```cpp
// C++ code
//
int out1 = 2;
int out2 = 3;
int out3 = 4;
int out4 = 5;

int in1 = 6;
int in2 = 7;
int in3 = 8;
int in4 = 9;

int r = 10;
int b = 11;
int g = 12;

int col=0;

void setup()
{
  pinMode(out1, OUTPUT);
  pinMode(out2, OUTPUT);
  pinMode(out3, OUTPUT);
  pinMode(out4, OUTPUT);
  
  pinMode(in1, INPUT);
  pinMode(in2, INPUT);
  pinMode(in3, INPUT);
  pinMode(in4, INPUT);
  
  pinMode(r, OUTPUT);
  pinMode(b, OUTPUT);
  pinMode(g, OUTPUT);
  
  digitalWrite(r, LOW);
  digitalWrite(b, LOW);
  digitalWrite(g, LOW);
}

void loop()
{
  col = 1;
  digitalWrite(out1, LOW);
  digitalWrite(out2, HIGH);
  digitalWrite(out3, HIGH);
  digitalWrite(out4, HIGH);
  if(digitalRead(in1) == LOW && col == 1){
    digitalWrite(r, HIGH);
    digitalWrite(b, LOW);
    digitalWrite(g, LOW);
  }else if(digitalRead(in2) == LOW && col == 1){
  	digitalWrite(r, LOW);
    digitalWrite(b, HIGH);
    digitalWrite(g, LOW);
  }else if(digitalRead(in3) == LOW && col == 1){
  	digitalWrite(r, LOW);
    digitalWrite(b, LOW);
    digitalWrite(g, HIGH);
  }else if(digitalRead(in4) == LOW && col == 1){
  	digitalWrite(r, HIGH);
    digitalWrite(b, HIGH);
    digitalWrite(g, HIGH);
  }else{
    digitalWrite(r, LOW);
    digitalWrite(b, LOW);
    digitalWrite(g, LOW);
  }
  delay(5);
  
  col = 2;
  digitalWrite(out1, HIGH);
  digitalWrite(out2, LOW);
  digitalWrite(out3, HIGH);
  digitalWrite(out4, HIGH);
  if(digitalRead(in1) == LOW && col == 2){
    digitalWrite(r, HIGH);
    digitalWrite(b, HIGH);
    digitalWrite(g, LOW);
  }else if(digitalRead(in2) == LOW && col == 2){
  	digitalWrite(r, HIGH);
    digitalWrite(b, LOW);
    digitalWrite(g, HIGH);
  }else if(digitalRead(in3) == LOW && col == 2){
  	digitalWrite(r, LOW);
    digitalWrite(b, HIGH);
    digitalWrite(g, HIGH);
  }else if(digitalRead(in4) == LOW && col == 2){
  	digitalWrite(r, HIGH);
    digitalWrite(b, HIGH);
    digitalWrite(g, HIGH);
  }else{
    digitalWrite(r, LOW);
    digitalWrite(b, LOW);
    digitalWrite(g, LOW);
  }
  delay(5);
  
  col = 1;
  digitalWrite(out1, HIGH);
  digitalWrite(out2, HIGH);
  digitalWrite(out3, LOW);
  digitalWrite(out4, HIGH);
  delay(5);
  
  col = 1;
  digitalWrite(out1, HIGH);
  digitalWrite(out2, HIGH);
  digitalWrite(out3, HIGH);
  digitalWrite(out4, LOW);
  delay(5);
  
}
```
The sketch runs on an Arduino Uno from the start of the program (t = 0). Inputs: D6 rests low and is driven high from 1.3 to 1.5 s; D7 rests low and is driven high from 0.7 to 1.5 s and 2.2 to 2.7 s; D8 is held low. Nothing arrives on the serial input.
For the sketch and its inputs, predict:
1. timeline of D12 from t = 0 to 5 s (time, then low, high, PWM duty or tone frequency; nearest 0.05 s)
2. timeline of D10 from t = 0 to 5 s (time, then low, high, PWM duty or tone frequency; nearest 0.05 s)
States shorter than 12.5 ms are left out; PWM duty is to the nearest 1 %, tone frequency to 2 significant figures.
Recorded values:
0 s low; 1.3 s high; 1.5 s low
0 s high; 1.3 s low; 1.5 s high
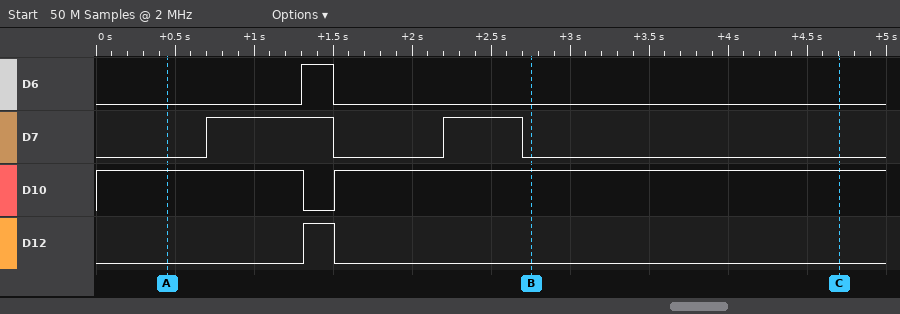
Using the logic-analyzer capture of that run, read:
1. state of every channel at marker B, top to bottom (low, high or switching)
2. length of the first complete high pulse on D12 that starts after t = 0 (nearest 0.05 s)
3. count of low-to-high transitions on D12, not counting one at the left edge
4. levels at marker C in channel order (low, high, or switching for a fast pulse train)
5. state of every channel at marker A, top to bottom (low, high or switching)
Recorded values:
D6 low, D7 low, D10 high, D12 low
0.20 s
1
D6 low, D7 low, D10 high, D12 low
D6 low, D7 low, D10 high, D12 low
